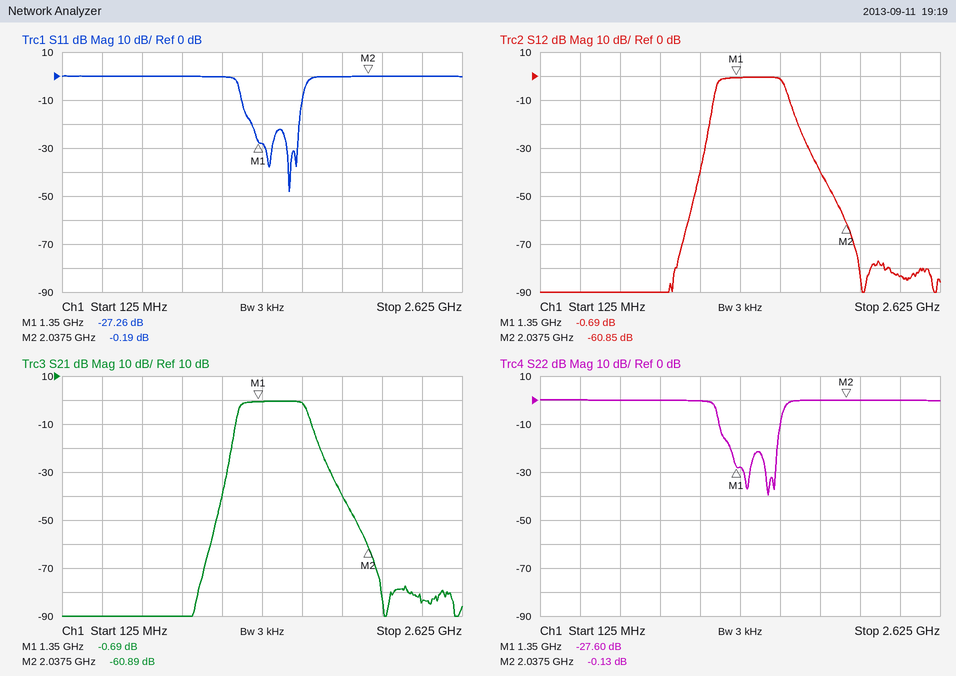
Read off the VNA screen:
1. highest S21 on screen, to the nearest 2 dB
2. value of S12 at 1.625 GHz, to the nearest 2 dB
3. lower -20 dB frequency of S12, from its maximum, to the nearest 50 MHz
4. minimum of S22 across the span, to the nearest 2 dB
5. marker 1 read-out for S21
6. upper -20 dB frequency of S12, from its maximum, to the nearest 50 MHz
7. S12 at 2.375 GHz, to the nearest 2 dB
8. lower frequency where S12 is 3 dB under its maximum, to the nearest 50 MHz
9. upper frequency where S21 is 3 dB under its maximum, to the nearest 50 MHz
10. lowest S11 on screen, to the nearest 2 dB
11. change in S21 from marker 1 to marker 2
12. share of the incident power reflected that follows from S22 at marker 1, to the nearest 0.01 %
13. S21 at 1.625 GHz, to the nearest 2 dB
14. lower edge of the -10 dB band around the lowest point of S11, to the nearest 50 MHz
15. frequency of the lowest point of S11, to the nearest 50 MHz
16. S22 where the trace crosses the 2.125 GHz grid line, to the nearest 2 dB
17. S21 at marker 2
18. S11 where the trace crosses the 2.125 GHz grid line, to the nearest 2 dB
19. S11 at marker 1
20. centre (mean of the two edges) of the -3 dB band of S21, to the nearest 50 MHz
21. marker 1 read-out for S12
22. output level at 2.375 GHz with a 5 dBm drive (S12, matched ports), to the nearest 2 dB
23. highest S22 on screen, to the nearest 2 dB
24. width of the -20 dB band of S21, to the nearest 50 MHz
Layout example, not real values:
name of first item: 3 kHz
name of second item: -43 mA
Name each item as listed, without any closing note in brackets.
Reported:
highest S21 on screen, to the nearest 2 dB: 0 dB
value of S12 at 1.625 GHz, to the nearest 2 dB: -2 dB
lower -20 dB frequency of S12, from its maximum, to the nearest 50 MHz: 1.20 GHz
minimum of S22 across the span, to the nearest 2 dB: -40 dB
marker 1 read-out for S21: -0.69 dB
upper -20 dB frequency of S12, from its maximum, to the nearest 50 MHz: 1.75 GHz
S12 at 2.375 GHz, to the nearest 2 dB: -84 dB
lower frequency where S12 is 3 dB under its maximum, to the nearest 50 MHz: 1.25 GHz
upper frequency where S21 is 3 dB under its maximum, to the nearest 50 MHz: 1.65 GHz
lowest S11 on screen, to the nearest 2 dB: -48 dB
change in S21 from marker 1 to marker 2: -60.20 dB
share of the incident power reflected that follows from S22 at marker 1, to the nearest 0.01 %: 0.17 %
S21 at 1.625 GHz, to the nearest 2 dB: -2 dB
lower edge of the -10 dB band around the lowest point of S11, to the nearest 50 MHz: 1.25 GHz
frequency of the lowest point of S11, to the nearest 50 MHz: 1.55 GHz
S22 where the trace crosses the 2.125 GHz grid line, to the nearest 2 dB: 0 dB
S21 at marker 2: -60.89 dB
S11 where the trace crosses the 2.125 GHz grid line, to the nearest 2 dB: 0 dB
S11 at marker 1: -27.26 dB
centre (mean of the two edges) of the -3 dB band of S21, to the nearest 50 MHz: 1.45 GHz
marker 1 read-out for S12: -0.69 dB
output level at 2.375 GHz with a 5 dBm drive (S12, matched ports), to the nearest 2 dB: -78 dBm
highest S22 on screen, to the nearest 2 dB: 0 dB
width of the -20 dB band of S21, to the nearest 50 MHz: 550 MHz
